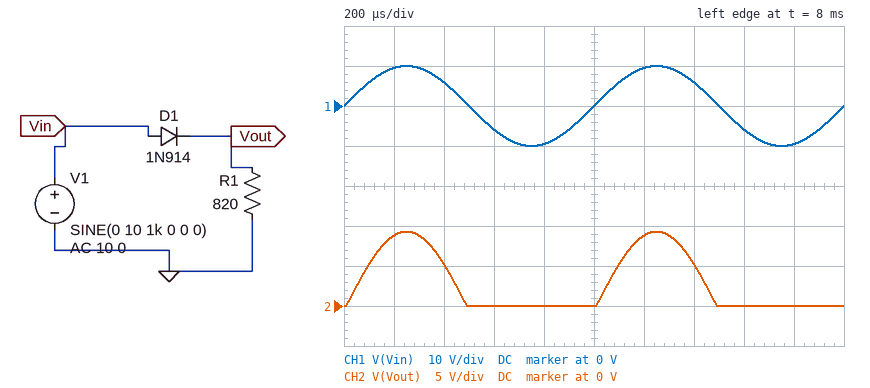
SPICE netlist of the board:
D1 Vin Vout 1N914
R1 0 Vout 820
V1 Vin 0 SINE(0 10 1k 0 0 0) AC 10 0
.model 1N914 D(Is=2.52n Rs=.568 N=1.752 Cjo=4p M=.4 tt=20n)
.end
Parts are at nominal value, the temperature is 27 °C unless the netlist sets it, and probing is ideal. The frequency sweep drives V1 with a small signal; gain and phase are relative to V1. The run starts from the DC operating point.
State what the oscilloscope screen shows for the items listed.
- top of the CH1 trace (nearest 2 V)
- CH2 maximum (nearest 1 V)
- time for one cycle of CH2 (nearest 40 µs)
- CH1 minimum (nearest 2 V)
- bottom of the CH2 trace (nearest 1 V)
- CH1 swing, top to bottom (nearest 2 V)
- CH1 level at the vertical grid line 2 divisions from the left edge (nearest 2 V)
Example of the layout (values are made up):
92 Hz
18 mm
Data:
10 V
9 V
1.00 ms
-10 V
0 V
20 V
6 V
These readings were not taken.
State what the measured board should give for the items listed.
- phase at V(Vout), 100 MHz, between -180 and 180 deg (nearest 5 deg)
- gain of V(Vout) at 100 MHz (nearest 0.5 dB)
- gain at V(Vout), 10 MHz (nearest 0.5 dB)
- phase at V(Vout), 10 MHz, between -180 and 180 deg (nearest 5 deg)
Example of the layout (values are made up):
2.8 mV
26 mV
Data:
25 deg
-1.0 dB
-14.0 dB
80 deg
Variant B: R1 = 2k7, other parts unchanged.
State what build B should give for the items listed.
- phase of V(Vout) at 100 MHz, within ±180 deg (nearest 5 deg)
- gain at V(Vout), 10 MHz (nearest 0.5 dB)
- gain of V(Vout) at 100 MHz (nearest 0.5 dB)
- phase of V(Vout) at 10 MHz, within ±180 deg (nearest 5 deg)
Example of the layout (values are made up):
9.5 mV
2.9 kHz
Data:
10 deg
-5.0 dB
0 dB
55 deg
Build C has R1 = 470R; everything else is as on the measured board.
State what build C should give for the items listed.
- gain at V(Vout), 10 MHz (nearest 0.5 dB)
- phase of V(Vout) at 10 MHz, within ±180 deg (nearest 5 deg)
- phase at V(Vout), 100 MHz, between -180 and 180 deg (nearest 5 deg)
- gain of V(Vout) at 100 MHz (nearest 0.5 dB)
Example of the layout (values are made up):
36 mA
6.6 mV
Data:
-18.5 dB
85 deg
40 deg
-2.5 dB
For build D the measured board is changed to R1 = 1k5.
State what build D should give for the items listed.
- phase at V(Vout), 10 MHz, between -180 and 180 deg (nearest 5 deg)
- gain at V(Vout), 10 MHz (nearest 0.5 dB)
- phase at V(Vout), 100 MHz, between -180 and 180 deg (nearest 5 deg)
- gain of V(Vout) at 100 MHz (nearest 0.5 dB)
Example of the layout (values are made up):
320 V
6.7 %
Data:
70 deg
-9.0 dB
15 deg
-0.5 dB
